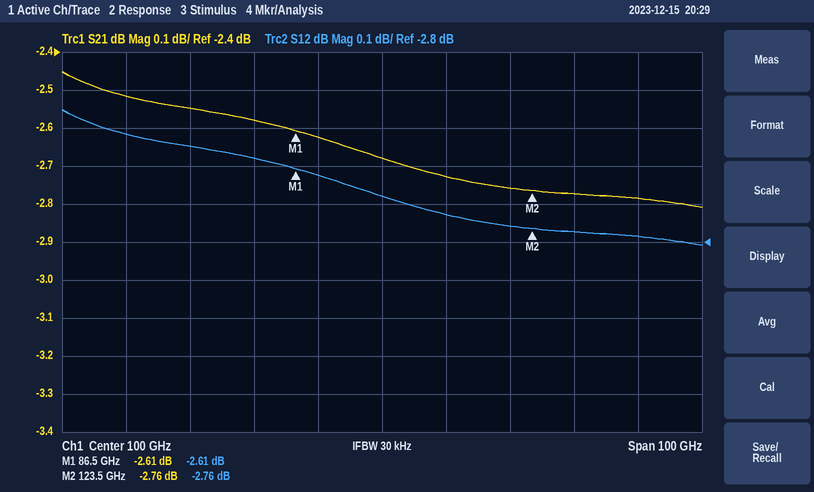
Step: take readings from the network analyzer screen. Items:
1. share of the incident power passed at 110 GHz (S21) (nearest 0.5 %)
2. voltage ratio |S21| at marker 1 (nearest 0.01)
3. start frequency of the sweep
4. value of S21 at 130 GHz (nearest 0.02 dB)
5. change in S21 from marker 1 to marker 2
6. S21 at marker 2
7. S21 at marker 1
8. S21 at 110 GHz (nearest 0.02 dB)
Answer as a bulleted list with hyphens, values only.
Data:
- 53.5 %
- 0.74
- 50 GHz
- -2.78 dB
- -0.15 dB
- -2.76 dB
- -2.61 dB
- -2.72 dB
